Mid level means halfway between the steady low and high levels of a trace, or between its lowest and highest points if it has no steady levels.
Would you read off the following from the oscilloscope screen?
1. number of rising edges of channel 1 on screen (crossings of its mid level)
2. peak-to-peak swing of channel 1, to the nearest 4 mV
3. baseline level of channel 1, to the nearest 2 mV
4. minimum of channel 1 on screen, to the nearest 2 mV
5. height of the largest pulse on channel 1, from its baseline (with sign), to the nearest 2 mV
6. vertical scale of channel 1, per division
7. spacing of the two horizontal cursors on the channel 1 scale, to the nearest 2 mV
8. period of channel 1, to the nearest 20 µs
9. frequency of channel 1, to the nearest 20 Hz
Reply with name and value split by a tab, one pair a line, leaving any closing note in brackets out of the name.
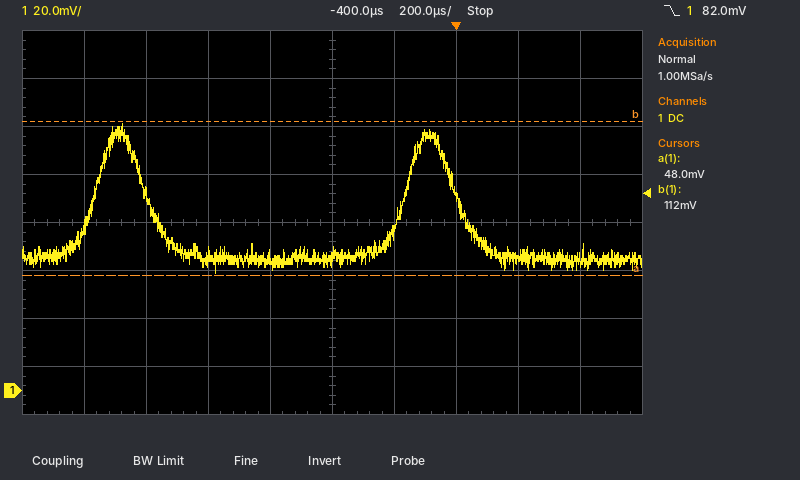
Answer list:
number of rising edges of channel 1 on screen	2
peak-to-peak swing of channel 1, to the nearest 4 mV	64 mV
baseline level of channel 1, to the nearest 2 mV	56 mV
minimum of channel 1 on screen, to the nearest 2 mV	48 mV
height of the largest pulse on channel 1, from its baseline (with sign), to the nearest 2 mV	+56 mV
vertical scale of channel 1, per division	20 mV
spacing of the two horizontal cursors on the channel 1 scale, to the nearest 2 mV	64 mV
period of channel 1, to the nearest 20 µs	1.00 ms
frequency of channel 1, to the nearest 20 Hz	1.00 kHz
